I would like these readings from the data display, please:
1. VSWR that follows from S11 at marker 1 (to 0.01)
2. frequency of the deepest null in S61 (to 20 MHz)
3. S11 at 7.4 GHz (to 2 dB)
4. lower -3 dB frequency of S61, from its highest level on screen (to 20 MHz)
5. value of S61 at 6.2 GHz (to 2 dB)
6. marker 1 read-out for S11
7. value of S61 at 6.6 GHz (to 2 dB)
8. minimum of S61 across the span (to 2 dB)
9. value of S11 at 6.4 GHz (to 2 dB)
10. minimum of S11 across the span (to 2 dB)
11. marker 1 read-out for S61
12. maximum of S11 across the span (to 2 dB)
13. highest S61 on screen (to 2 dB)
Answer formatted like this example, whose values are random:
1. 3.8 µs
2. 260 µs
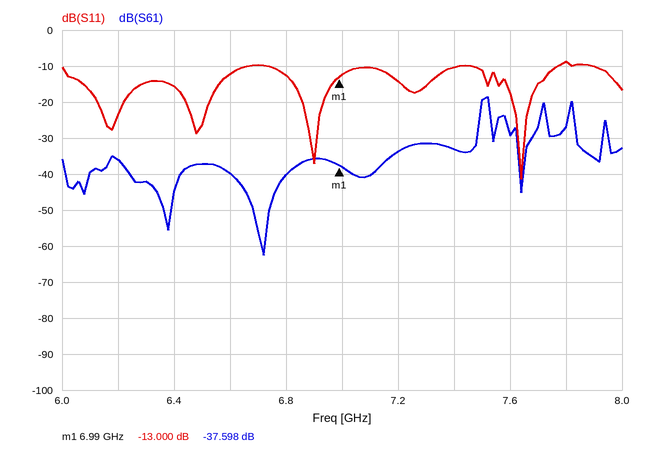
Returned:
1. 1.58
2. 6.72 GHz
3. -10 dB
4. 7.50 GHz
5. -36 dB
6. -13.000 dB
7. -40 dB
8. -62 dB
9. -16 dB
10. -42 dB
11. -37.598 dB
12. -8 dB
13. -18 dB
